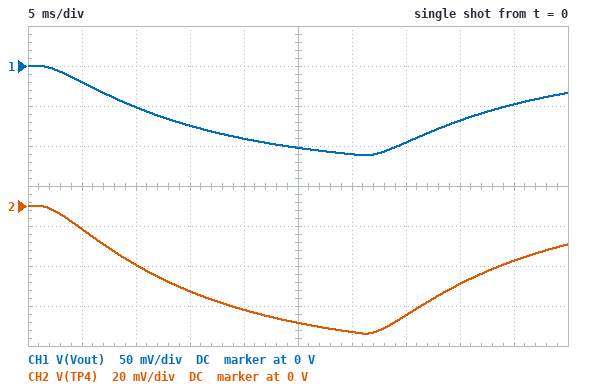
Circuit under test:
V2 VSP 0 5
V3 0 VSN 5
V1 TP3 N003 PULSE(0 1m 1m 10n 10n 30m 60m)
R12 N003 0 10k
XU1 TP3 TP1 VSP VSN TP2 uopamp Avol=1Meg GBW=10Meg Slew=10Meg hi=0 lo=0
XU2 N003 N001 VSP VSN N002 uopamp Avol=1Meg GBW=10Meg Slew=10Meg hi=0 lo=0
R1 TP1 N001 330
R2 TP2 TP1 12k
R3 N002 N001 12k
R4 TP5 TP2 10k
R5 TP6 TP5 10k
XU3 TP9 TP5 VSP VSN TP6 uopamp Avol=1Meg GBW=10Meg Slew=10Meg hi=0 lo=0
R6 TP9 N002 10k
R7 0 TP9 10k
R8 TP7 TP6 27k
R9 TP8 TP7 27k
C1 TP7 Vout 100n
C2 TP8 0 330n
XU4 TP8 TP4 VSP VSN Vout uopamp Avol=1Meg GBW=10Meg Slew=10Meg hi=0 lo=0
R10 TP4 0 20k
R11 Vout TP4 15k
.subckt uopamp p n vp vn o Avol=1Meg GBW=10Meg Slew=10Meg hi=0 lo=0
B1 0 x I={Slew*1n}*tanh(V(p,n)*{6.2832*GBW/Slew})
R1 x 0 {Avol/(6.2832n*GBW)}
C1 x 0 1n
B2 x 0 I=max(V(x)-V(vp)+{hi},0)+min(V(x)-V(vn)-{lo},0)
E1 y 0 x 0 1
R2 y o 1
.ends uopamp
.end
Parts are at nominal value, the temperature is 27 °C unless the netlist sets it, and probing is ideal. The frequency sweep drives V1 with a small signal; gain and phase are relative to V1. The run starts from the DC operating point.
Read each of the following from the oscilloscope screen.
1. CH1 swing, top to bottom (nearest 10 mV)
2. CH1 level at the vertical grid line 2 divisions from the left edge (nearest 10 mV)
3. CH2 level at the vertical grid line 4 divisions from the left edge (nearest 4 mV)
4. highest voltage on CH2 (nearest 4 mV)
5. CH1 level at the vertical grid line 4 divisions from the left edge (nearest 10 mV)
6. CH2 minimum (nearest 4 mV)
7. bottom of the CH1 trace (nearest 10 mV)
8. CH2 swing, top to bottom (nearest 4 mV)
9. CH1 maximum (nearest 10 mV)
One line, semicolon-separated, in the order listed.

110 mV; -50 mV; -52 mV; 0 V; -90 mV; -64 mV; -110 mV; 64 mV; 0 V
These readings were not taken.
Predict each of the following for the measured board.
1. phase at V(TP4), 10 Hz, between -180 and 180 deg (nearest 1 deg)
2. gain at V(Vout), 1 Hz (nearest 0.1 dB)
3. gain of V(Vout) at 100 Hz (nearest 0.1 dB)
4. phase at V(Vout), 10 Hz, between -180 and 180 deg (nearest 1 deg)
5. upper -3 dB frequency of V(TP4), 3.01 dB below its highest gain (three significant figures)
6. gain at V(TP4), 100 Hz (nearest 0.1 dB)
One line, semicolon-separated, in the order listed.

132 deg; 42.2 dB; 19.9 dB; 132 deg; 11.1 Hz; 15.0 dB
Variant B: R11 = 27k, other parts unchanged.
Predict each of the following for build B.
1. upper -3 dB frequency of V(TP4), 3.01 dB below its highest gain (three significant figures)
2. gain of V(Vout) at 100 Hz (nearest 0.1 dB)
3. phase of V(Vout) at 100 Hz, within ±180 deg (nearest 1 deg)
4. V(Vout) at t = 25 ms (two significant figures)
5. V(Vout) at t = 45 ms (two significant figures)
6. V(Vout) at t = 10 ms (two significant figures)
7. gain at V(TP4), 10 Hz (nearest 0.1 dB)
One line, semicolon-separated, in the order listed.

12.7 Hz; 23.0 dB; 46 deg; -140 mV; -60 mV; -75 mV; 35.3 dB
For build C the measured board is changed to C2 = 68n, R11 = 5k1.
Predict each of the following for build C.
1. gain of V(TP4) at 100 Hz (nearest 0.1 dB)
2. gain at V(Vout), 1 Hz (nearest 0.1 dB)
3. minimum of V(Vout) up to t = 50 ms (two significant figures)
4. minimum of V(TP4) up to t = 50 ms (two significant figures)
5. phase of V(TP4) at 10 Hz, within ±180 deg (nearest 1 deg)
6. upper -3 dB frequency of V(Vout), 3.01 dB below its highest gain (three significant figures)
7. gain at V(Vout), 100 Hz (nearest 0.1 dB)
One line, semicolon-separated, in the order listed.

30.9 dB; 39.3 dB; -98 mV; -78 mV; 169 deg; 74.9 Hz; 32.9 dB
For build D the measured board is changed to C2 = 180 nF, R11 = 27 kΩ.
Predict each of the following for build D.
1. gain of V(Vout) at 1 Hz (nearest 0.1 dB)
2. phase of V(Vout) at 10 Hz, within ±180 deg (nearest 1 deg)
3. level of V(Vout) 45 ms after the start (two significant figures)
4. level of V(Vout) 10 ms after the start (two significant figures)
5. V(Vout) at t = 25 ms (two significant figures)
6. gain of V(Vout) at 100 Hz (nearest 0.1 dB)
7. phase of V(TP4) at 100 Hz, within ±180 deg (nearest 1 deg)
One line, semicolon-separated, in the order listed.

44.8 dB; 158 deg; -5.5 mV; -140 mV; -170 mV; 29.7 dB; 42 deg
